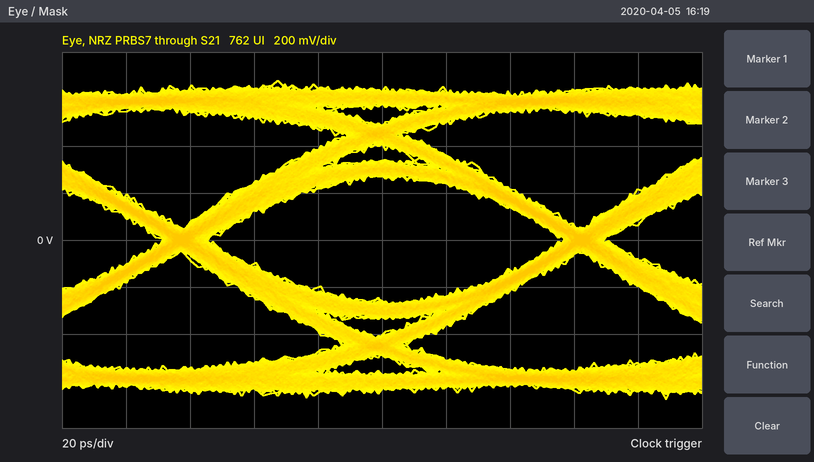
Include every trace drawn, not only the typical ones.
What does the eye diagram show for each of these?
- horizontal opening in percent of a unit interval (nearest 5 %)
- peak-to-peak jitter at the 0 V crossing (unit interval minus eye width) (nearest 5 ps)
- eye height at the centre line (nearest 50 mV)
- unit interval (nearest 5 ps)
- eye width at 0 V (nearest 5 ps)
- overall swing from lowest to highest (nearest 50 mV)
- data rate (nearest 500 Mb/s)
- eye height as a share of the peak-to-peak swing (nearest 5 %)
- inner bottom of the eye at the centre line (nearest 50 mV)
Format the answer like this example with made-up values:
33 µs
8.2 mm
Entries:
90 %
15 ps
550 mV
125 ps
110 ps
1.35 V
8.0 Gb/s
40 %
-250 mV
